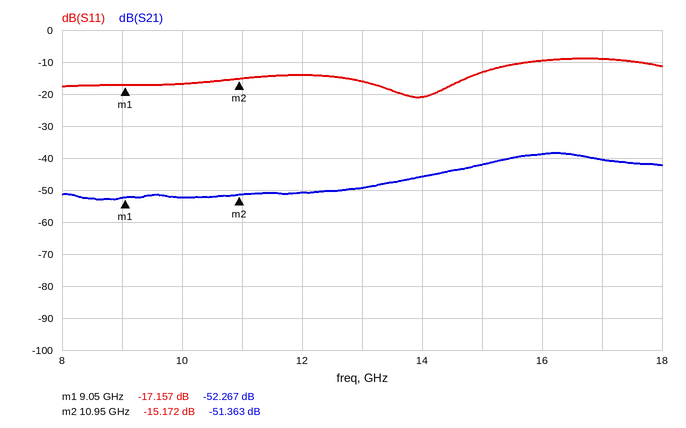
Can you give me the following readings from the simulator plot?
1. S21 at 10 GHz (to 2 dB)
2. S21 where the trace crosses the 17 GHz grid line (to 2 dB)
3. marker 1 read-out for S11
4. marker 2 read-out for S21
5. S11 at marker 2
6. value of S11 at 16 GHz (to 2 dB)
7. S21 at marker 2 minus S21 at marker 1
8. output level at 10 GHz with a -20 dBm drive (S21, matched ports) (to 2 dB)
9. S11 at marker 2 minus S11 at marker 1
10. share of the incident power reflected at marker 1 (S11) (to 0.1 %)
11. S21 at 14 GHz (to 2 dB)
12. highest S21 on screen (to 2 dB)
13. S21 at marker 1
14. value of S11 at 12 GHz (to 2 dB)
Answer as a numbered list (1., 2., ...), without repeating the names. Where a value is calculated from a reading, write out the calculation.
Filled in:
1. -52 dB
2. -40 dB
3. -17.157 dB
4. -51.363 dB
5. -15.172 dB
6. -10 dB
7. -51.363 − (-52.267) = 0.904 dB
8. -20 dBm + (-52 dB) = -72 dBm
9. -15.172 − (-17.157) = 1.985 dB
10. 10^(-17.157/10) ≈ 1.9 %
11. -46 dB
12. -38 dB
13. -52.267 dB
14. -14 dB
